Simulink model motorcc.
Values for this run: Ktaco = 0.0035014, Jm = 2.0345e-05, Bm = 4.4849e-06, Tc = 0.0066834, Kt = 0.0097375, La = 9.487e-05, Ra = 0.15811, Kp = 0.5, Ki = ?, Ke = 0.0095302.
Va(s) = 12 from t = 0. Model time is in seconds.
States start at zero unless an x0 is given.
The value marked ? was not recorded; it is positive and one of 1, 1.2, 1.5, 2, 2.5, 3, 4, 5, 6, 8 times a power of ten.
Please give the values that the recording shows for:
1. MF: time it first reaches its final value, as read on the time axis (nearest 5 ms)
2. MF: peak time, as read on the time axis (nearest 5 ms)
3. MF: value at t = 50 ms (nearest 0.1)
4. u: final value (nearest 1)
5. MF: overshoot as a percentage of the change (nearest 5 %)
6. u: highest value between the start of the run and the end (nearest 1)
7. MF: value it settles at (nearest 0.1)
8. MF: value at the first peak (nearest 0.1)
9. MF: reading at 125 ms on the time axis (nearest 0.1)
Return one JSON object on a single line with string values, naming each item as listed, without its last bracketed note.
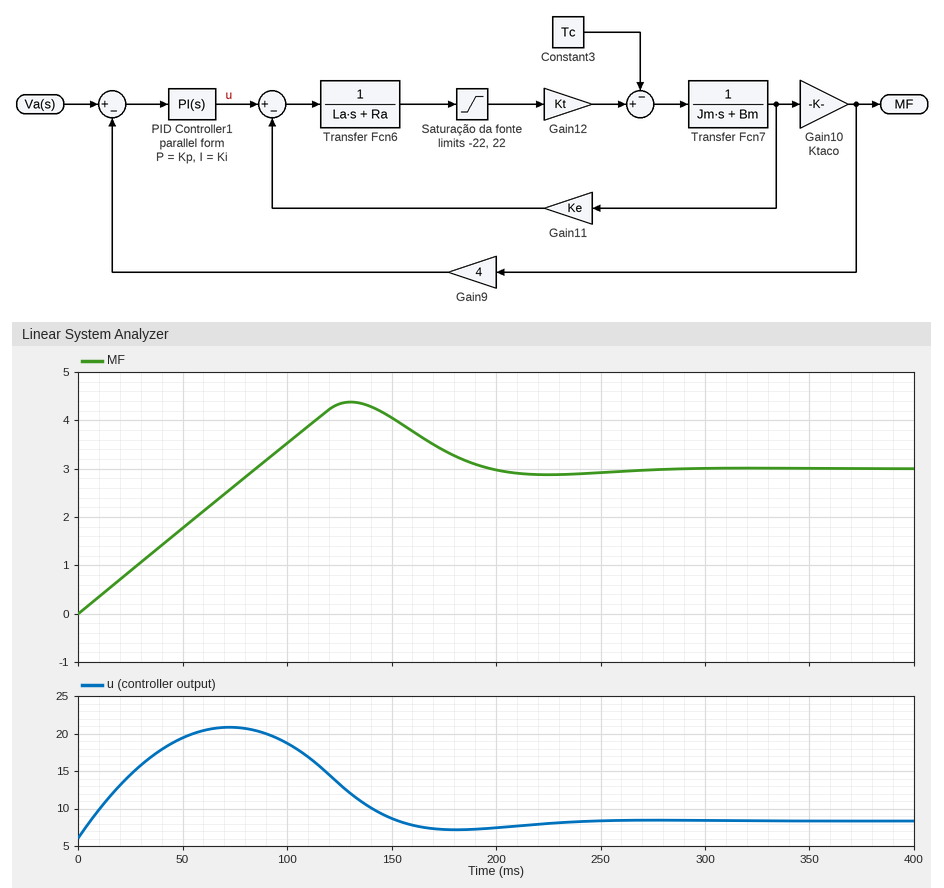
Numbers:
{"MF: time it first reaches its final value, as read on the time axis": "85 ms", "MF: peak time, as read on the time axis": "130 ms", "MF: value at t = 50 ms": "1.8", "u: final value": "8", "MF: overshoot as a percentage of the change": "45 %", "u: highest value between the start of the run and the end": "21", "MF: value it settles at": "3.0", "MF: value at the first peak": "4.4", "MF: reading at 125 ms on the time axis": "4.3"}
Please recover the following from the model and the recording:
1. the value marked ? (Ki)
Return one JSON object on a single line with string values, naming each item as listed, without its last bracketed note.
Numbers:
{"the value marked ?": "40"}
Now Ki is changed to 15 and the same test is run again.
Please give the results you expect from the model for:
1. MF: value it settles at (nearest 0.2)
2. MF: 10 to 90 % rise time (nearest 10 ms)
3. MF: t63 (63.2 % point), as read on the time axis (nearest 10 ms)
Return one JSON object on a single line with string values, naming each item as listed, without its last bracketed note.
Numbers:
{"MF: value it settles at": "3.0", "MF: 10 to 90 % rise time": "80 ms", "MF: t63 (63.2 % point), as read on the time axis": "50 ms"}
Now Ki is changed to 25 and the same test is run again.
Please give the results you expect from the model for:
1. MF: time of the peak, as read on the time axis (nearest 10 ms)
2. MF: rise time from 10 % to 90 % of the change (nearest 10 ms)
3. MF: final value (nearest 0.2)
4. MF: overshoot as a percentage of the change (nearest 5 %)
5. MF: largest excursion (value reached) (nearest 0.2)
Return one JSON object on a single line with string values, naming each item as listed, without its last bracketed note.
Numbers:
{"MF: time of the peak, as read on the time axis": "120 ms", "MF: rise time from 10 % to 90 % of the change": "70 ms", "MF: final value": "3.0", "MF: overshoot as a percentage of the change": "20 %", "MF: largest excursion (value reached)": "3.6"}
